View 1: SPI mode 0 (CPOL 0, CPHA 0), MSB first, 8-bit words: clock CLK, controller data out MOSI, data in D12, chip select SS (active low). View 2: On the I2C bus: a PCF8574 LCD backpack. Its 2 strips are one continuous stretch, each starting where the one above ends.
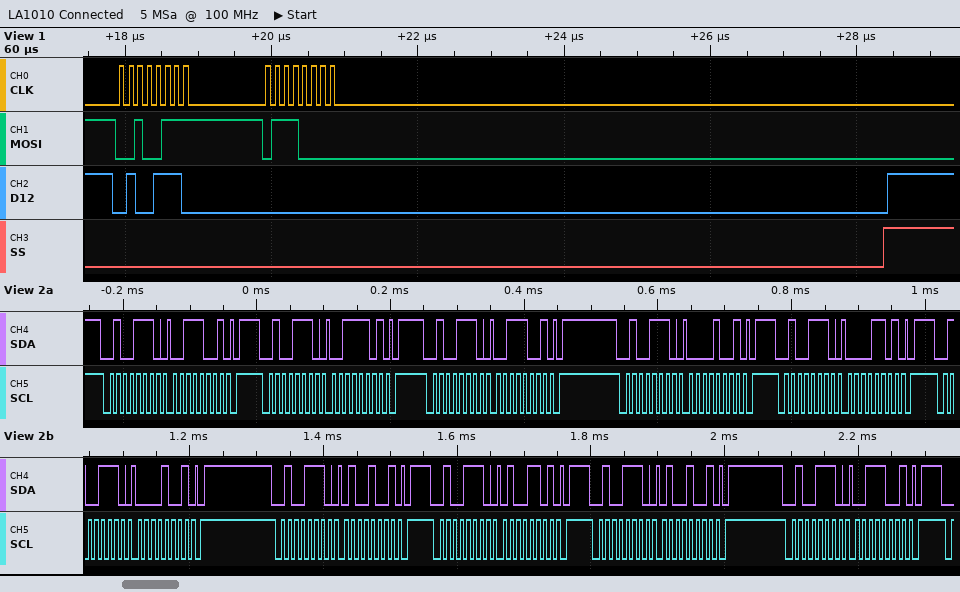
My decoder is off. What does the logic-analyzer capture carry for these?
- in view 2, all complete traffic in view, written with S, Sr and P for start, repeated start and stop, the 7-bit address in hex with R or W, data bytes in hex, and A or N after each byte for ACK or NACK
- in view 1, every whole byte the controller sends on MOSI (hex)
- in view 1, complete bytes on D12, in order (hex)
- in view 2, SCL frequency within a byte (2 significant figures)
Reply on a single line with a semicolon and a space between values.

S 27W A 39 A P S 27W A 3D A P S 27W A 39 A P S 27W A 09 A P S 27W A 0D A P S 27W A 09 A P S 27W A 49 A P S 27W A 4D A P S 27W A 49 A P S 27W A 39 A P; 27 70; 4E 00; 100 kHz
